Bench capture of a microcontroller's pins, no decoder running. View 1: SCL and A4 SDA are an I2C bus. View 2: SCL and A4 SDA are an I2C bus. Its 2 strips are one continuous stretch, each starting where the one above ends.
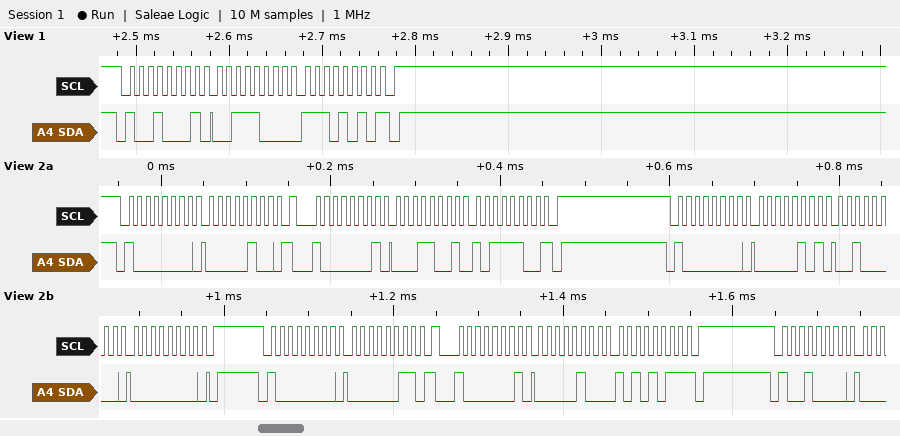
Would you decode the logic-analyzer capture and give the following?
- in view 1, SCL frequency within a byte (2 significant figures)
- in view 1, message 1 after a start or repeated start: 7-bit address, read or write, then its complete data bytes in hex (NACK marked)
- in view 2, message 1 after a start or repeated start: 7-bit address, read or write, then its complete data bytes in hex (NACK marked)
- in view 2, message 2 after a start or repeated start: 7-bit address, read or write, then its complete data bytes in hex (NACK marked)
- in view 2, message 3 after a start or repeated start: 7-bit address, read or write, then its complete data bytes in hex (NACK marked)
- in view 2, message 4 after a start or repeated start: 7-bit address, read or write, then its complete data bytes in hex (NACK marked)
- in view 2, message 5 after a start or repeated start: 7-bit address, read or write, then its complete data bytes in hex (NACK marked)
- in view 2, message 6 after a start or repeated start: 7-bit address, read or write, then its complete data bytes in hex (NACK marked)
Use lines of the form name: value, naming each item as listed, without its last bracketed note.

in view 1, SCL frequency within a byte: 100 kHz
in view 1, message 1 after a start or repeated start: 7-bit address, read or write, then its complete data bytes in hex: 0x48 read: 38 EA NACK
in view 2, message 1 after a start or repeated start: 7-bit address, read or write, then its complete data bytes in hex: 0x40 write: 04
in view 2, message 2 after a start or repeated start: 7-bit address, read or write, then its complete data bytes in hex: 0x40 read: 19 BC NACK
in view 2, message 3 after a start or repeated start: 7-bit address, read or write, then its complete data bytes in hex: 0x40 write: 05 20 00
in view 2, message 4 after a start or repeated start: 7-bit address, read or write, then its complete data bytes in hex: 0x40 write: 03
in view 2, message 5 after a start or repeated start: 7-bit address, read or write, then its complete data bytes in hex: 0x40 read: 04 AB NACK
in view 2, message 6 after a start or repeated start: 7-bit address, read or write, then its complete data bytes in hex: 0x48 write
